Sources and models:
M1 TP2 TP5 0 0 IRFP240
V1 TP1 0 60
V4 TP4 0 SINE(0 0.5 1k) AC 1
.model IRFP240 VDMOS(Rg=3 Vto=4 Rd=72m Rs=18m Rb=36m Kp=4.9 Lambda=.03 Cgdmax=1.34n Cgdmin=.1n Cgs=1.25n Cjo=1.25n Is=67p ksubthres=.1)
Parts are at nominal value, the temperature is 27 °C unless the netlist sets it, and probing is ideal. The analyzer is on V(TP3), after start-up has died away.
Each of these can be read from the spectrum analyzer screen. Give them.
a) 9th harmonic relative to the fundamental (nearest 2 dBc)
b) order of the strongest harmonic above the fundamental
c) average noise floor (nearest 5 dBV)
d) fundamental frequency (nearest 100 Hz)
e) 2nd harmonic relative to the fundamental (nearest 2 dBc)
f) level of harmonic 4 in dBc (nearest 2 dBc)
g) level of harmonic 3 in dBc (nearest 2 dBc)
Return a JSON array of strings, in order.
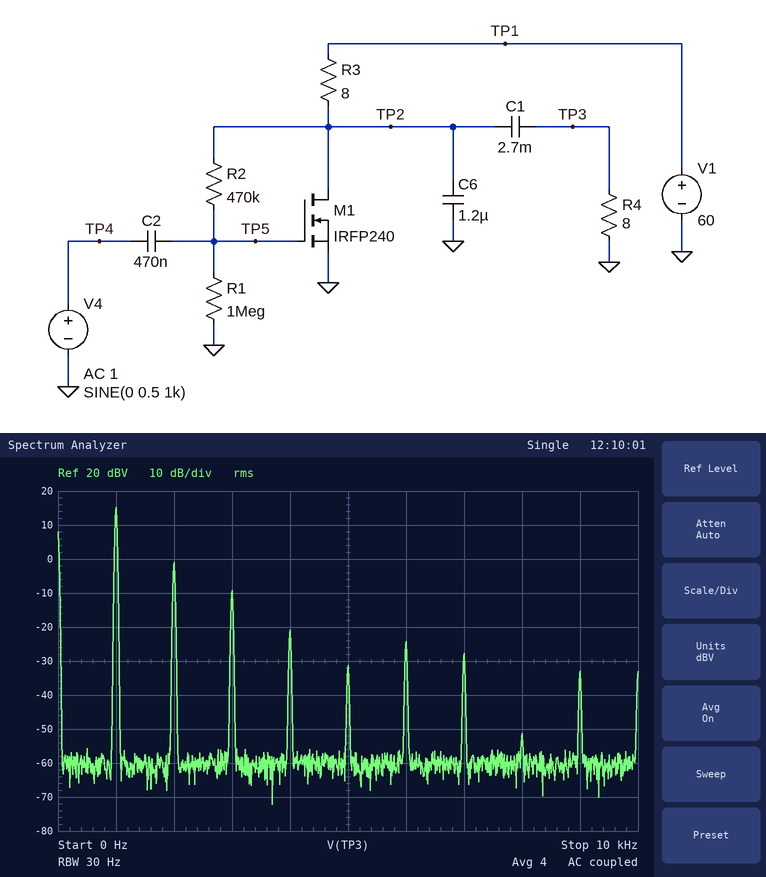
["-48 dBc", "2", "-60 dBV", "1.0 kHz", "-16 dBc", "-36 dBc", "-24 dBc"]
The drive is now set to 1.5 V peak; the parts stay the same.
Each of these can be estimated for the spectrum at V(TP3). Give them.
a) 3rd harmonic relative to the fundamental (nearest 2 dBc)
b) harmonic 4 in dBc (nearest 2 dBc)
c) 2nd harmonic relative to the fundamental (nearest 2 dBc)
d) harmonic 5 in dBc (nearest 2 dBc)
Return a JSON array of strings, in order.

["-22 dBc", "-22 dBc", "-6 dBc", "-28 dBc"]
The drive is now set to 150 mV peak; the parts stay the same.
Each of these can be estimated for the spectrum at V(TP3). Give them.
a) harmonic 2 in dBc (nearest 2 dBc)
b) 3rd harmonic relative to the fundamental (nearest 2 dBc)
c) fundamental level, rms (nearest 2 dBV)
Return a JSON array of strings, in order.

["-36 dBc", "-56 dBc", "6 dBV"]
